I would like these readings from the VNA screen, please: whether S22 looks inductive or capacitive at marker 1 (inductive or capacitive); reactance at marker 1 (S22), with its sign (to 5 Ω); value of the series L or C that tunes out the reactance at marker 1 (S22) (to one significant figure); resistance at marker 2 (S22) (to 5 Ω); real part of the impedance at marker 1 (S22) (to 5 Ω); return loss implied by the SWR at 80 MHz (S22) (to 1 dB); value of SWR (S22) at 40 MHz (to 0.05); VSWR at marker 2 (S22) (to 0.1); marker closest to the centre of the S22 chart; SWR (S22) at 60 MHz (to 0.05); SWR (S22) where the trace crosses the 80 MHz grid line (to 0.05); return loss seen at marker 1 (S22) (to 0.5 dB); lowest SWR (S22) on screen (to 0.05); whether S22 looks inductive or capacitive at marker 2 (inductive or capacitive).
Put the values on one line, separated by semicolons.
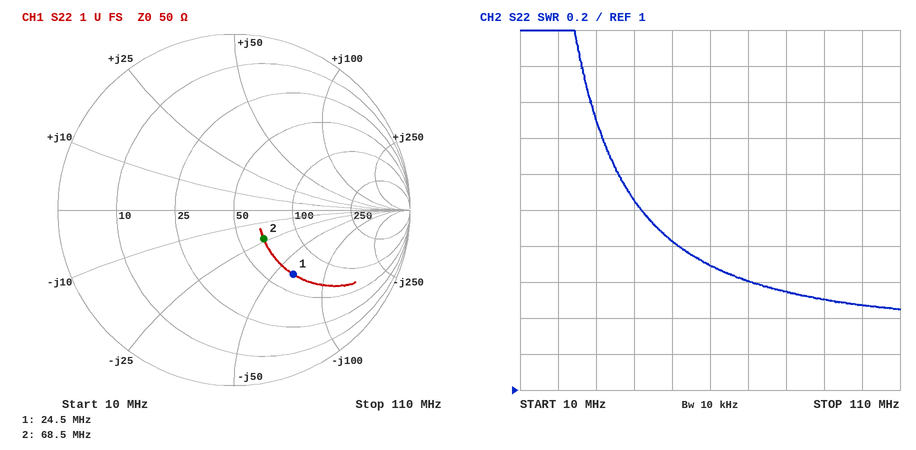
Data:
capacitive; -65 Ω; 400 nH; 65 Ω; 65 Ω; 13 dB; 2.05; 1.6; marker 2; 1.70; 1.55; 6.0 dB; 1.45; capacitive
